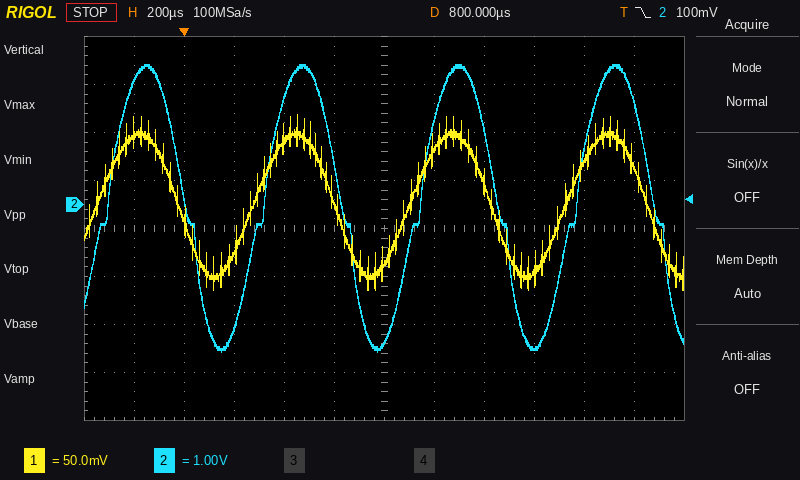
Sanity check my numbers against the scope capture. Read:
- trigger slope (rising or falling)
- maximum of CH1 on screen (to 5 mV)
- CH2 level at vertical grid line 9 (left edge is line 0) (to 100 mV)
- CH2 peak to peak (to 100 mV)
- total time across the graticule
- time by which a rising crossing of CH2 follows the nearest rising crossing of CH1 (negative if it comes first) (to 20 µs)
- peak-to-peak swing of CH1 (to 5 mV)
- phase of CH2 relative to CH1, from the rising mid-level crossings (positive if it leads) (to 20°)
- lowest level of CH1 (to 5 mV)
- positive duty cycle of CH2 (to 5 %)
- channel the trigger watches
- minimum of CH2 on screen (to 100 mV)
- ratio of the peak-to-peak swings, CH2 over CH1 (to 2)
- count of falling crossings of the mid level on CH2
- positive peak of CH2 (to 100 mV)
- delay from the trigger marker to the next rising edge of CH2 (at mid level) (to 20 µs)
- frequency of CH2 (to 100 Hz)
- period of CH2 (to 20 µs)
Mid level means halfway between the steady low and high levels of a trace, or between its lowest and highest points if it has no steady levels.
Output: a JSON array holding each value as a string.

["falling", "95 mV", "-3.0 V", "6.0 V", "2.4 ms", "+40 µs", "185 mV", "-20°", "-90 mV", "50 %", "CH2", "-3.1 V", "32", "4", "2.9 V", "320 µs", "1.6 kHz", "620 µs"]
